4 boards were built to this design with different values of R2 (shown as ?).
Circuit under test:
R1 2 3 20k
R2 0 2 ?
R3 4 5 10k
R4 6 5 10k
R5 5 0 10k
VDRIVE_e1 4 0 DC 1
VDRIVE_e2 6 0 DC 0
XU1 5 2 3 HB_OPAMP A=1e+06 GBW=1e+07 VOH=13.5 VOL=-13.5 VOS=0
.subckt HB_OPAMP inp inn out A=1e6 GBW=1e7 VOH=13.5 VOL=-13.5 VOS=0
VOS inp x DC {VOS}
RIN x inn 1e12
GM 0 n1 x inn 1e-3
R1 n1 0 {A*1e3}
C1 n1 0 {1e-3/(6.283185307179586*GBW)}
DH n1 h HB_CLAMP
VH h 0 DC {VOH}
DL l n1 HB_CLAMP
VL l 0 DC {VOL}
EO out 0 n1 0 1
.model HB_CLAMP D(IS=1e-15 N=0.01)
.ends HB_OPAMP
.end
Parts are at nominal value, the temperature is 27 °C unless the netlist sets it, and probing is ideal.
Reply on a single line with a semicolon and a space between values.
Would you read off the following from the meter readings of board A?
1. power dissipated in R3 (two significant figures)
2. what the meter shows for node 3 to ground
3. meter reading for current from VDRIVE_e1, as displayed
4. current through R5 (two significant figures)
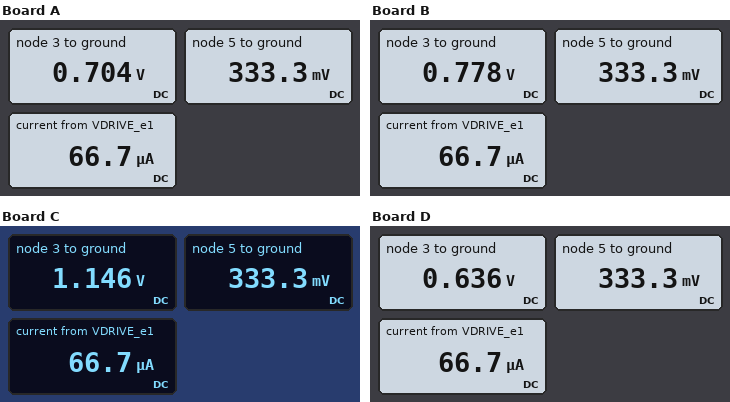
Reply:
44 µW; 0.704 V; 66.7 µA; 33 µA
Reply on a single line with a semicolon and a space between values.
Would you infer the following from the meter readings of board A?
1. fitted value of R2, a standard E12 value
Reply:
18 kΩ
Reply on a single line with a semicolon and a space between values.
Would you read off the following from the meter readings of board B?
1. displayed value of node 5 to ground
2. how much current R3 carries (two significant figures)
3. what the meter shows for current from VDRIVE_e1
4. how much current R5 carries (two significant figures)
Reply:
333.3 mV; 67 µA; 66.7 µA; 33 µA
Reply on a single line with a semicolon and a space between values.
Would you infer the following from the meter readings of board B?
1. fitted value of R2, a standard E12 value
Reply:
15 kΩ
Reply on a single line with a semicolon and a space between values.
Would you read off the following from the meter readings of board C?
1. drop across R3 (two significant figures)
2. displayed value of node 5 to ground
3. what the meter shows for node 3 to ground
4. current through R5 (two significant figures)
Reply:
670 mV; 333.3 mV; 1.146 V; 33 µA
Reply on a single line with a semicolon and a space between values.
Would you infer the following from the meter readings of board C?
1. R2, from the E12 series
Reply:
8.2 kΩ
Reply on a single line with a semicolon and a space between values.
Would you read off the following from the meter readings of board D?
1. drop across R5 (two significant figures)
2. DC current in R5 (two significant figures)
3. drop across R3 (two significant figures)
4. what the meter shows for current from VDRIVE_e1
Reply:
330 mV; 33 µA; 670 mV; 66.7 µA
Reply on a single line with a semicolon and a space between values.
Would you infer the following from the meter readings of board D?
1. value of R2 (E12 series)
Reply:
22 kΩ
